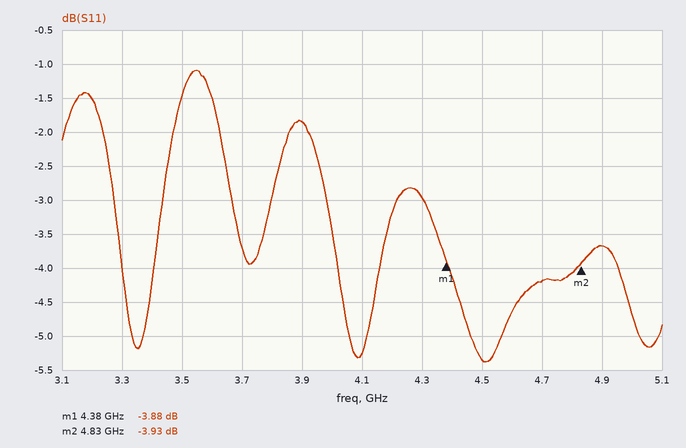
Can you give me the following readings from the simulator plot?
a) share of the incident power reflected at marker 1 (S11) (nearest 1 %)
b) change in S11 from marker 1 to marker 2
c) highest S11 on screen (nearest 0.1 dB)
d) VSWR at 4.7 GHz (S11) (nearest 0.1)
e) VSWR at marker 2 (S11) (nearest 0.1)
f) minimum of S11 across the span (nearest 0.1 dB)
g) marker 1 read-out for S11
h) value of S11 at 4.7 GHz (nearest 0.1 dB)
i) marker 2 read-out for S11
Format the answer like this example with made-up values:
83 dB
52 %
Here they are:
41 %
-0.05 dB
-1.1 dB
4.2
4.5
-5.4 dB
-3.88 dB
-4.2 dB
-3.93 dB
